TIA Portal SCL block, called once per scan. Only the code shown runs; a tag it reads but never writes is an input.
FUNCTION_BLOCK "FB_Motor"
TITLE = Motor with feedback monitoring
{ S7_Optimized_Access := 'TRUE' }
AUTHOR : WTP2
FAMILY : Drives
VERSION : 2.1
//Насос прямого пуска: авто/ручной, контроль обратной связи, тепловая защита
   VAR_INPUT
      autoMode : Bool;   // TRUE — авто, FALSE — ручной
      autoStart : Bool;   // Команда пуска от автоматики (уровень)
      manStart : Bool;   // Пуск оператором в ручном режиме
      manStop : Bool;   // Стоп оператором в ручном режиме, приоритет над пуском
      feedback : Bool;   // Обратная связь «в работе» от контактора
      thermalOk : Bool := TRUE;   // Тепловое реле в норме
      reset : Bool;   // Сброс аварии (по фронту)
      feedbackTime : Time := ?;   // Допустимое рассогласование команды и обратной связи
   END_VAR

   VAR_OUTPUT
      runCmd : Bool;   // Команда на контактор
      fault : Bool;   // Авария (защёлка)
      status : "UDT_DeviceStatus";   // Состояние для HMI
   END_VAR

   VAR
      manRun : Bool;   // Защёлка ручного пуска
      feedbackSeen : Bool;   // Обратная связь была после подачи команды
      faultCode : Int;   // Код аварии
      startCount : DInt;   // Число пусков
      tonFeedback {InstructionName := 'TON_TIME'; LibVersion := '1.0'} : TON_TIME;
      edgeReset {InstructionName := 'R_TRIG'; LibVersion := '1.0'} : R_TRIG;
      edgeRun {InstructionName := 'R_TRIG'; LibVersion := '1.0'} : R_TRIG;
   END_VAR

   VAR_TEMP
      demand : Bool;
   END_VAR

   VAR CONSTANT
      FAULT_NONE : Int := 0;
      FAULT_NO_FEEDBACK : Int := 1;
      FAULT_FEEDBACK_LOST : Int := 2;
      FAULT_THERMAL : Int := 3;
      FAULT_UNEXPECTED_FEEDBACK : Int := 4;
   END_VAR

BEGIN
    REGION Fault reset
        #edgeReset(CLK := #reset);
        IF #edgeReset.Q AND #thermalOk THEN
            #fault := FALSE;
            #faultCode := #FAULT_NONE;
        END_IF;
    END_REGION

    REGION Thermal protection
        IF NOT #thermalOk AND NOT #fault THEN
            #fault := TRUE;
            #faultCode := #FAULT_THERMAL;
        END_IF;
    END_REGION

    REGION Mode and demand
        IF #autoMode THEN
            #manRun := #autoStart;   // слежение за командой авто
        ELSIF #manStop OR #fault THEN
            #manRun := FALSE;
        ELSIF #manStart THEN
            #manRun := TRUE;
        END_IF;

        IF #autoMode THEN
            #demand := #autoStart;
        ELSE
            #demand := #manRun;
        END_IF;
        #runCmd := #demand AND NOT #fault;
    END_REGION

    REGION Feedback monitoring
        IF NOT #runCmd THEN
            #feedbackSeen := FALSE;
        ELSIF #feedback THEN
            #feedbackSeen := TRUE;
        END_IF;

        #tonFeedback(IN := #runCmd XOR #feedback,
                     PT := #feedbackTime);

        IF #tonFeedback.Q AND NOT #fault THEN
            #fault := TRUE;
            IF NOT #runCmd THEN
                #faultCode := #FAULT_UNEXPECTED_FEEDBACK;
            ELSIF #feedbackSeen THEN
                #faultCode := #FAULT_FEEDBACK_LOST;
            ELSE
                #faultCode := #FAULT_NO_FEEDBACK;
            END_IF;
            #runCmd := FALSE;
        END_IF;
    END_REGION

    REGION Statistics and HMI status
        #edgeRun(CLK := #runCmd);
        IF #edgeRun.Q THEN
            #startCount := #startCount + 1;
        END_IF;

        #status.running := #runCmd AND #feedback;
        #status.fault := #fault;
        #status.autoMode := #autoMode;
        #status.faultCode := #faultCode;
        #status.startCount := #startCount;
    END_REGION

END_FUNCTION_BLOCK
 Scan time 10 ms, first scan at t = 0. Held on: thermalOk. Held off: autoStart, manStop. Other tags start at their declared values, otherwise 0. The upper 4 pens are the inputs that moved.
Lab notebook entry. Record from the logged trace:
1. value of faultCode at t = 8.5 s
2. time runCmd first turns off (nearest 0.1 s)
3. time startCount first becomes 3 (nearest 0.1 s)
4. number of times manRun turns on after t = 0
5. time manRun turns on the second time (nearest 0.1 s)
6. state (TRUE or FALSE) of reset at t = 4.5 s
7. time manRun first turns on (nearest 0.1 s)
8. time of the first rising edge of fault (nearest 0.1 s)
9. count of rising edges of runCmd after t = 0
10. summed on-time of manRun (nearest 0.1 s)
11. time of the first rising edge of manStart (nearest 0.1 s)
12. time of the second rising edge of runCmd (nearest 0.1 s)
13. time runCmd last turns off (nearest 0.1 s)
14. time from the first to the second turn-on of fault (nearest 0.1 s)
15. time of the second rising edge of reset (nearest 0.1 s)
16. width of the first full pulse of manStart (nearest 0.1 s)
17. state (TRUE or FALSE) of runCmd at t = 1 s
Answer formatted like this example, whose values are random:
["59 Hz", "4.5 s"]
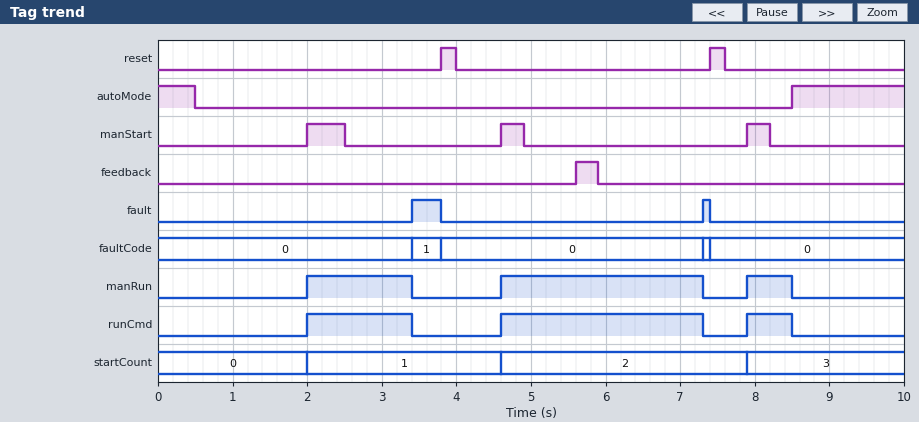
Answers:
["0", "3.4 s", "7.9 s", "3", "4.6 s", "FALSE", "2.0 s", "3.4 s", "3", "4.7 s", "2.0 s", "4.6 s", "8.5 s", "3.9 s", "7.4 s", "0.5 s", "FALSE"]
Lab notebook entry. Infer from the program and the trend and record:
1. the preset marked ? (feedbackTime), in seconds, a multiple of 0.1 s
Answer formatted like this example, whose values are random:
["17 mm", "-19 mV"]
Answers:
["1.4 s"]
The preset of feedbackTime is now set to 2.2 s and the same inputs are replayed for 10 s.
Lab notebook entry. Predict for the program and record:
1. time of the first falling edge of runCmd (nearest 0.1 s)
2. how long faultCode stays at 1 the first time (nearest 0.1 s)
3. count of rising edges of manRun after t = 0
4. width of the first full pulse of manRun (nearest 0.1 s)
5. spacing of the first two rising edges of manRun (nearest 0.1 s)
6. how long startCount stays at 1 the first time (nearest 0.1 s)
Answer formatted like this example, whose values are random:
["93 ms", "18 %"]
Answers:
["4.2 s", "3.2 s", "2", "2.2 s", "5.9 s", "5.9 s"]
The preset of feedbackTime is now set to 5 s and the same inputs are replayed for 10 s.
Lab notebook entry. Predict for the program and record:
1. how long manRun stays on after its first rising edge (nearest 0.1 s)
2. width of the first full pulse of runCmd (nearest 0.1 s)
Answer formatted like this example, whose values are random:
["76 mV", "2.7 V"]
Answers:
["6.5 s", "6.5 s"]
